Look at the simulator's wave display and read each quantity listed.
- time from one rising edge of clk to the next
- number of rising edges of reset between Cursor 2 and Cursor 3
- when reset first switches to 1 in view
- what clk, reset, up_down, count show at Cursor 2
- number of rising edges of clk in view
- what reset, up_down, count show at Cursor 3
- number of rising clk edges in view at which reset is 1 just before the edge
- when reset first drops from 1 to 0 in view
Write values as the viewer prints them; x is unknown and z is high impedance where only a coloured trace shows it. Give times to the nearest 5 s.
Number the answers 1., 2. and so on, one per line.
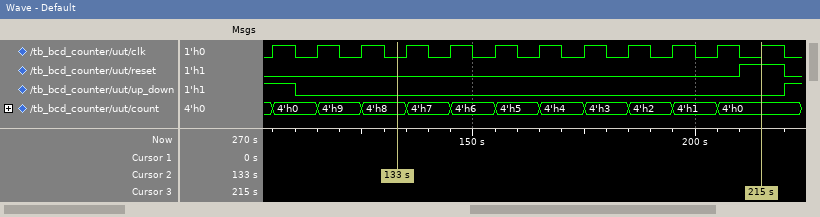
1. 10 s
2. 1
3. 210 s
4. clk=0, reset=0, up_down=0, count=4'h8
5. 12
6. reset=1, up_down=0, count=4'h0
7. 1
8. 220 s
